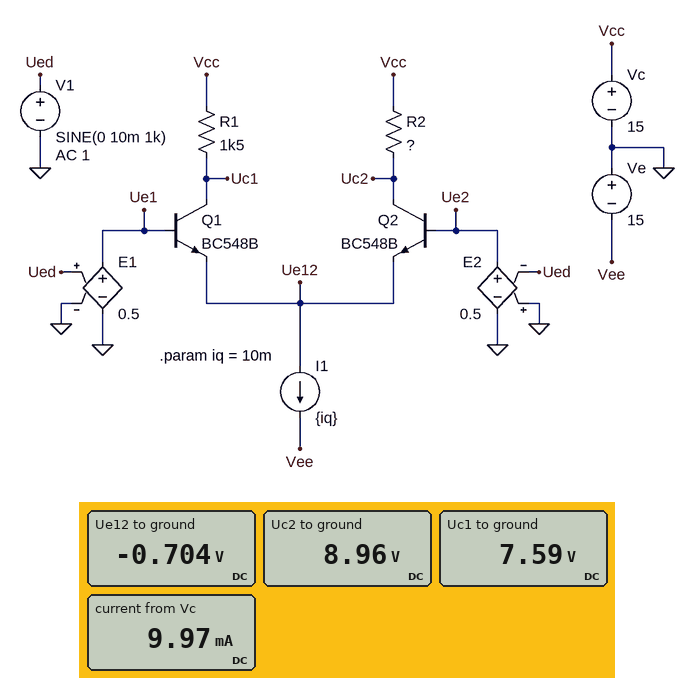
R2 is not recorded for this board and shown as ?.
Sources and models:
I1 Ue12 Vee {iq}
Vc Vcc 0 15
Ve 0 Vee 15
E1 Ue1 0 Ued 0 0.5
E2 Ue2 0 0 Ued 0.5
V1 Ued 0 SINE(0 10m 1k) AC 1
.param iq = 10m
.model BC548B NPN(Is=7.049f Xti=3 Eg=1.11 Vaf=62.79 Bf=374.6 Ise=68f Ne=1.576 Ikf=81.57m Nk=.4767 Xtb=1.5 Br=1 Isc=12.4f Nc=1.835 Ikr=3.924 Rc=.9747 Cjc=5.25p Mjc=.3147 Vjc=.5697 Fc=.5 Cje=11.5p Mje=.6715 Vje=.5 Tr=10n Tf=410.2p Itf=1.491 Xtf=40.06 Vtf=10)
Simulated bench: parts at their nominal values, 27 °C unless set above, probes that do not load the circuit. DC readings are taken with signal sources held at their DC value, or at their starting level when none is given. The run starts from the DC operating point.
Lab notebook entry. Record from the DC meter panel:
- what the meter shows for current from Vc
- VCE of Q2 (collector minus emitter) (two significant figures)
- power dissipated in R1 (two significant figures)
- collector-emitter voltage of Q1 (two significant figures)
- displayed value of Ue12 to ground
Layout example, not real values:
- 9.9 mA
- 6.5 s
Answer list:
- 9.97 mA
- 9.7 V
- 37 mW
- 8.3 V
- -0.704 V
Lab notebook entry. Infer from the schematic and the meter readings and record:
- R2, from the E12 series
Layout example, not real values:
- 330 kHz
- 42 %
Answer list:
- 1.2 kΩ
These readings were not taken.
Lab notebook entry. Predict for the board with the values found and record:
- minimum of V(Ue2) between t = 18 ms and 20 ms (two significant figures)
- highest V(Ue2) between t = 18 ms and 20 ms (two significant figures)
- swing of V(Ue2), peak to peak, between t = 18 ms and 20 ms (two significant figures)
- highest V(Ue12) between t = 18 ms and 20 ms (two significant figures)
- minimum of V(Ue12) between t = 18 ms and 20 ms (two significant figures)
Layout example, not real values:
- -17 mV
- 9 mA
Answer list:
- -5.0 mV
- 5.0 mV
- 10 mV
- -700 mV
- -700 mV
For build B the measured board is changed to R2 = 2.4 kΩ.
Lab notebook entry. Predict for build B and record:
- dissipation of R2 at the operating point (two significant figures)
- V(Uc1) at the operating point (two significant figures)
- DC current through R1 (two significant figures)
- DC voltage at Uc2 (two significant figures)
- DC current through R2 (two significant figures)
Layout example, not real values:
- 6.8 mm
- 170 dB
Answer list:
- 56 mW
- 7.3 V
- 5.1 mA
- 3.4 V
- 4.8 mA
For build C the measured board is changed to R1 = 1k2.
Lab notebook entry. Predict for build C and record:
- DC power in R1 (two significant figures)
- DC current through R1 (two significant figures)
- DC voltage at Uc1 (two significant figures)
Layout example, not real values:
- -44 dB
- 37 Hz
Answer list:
- 30 mW
- 5.0 mA
- 9.0 V
